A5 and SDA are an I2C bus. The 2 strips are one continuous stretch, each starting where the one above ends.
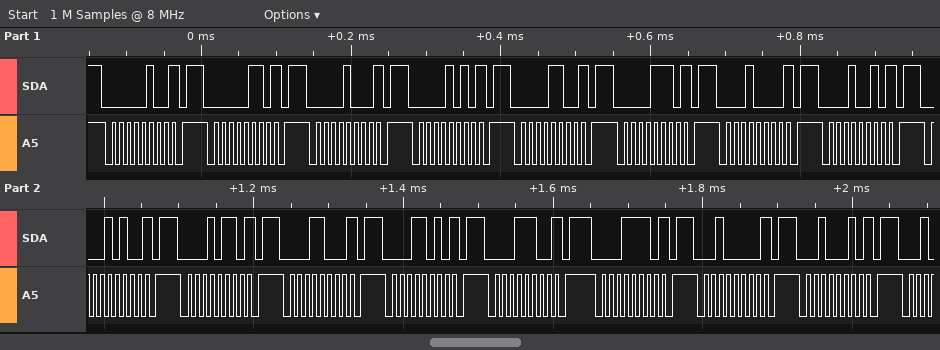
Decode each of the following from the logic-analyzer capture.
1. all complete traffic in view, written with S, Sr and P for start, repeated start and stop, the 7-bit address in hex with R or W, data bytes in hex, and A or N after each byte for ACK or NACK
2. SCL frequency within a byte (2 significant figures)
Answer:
S 02W N P S 03W N P S 04W N P S 05W N P S 06W N P S 07W N P S 08W N P S 09W N P S 0AW N P S 0BW N P S 0CW N P S 0DW N P S 0EW N P S 0FW N P S 10W N P S 11W N P
100 kHz
